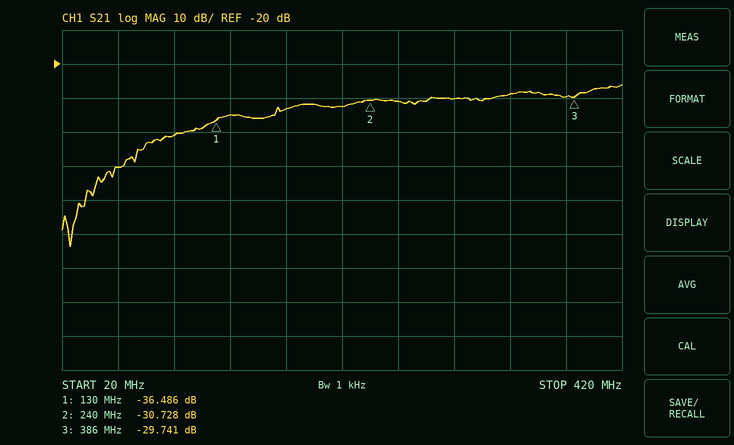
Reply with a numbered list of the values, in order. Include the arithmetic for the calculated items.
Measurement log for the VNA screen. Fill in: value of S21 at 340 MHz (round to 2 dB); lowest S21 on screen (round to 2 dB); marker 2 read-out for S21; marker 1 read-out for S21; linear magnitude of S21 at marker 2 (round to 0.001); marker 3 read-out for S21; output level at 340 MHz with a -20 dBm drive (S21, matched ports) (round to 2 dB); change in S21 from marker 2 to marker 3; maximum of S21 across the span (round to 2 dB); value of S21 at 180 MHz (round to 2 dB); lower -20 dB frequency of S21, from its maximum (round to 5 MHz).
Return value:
1. -28 dB
2. -74 dB
3. -30.728 dB
4. -36.486 dB
5. 10^(-30.728/20) ≈ 0.029
6. -29.741 dB
7. -20 dBm + (-28 dB) = -48 dBm
8. -29.741 − (-30.728) = 0.987 dB
9. -26 dB
10. -34 dB
11. 75 MHz
